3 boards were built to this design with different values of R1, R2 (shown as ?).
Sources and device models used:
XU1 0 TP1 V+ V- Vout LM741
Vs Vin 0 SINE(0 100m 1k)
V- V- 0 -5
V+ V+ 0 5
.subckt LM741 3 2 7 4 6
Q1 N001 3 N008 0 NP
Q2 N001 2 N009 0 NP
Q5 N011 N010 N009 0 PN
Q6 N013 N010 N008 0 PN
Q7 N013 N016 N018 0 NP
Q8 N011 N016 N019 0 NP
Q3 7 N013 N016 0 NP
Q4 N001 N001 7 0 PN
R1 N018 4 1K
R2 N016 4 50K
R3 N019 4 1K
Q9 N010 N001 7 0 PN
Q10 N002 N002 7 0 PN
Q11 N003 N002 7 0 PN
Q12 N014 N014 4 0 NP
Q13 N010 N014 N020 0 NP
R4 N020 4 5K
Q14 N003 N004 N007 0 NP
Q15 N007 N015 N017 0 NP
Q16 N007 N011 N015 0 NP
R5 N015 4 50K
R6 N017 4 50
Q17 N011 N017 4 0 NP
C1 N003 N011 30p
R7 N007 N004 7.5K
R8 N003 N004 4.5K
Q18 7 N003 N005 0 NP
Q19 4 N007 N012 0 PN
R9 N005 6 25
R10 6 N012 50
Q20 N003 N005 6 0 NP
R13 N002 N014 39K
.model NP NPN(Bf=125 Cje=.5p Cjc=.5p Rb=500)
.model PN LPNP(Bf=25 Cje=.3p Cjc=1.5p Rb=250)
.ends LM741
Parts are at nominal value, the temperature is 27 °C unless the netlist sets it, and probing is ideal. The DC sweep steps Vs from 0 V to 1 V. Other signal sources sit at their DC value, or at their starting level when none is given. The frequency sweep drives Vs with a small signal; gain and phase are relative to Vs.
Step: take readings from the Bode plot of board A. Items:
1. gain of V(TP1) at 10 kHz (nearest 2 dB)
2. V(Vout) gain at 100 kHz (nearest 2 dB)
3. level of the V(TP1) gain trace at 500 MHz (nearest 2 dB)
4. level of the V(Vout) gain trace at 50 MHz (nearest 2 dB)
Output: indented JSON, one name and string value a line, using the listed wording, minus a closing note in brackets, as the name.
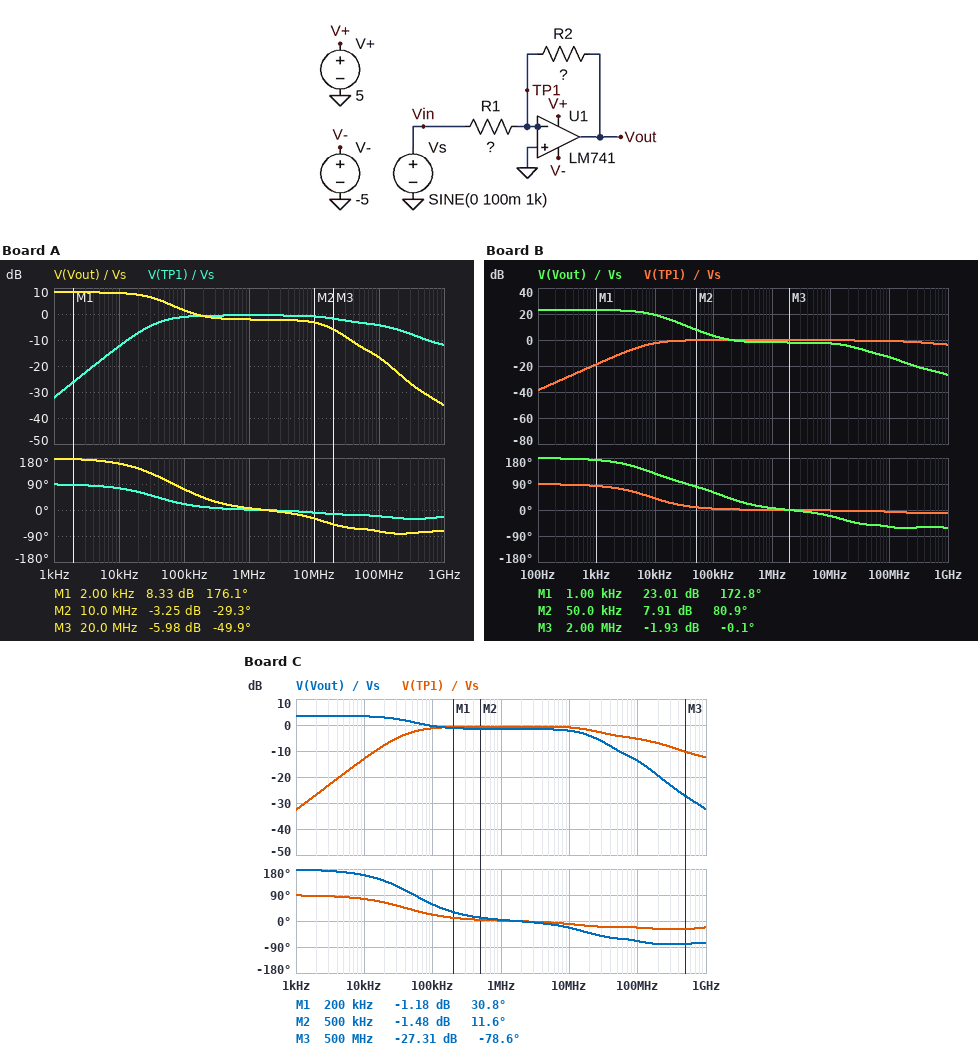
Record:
{
  "gain of V(TP1) at 10 kHz": "-12 dB",
  "V(Vout) gain at 100 kHz": "2 dB",
  "level of the V(TP1) gain trace at 500 MHz": "-10 dB",
  "level of the V(Vout) gain trace at 50 MHz": "-12 dB"
}
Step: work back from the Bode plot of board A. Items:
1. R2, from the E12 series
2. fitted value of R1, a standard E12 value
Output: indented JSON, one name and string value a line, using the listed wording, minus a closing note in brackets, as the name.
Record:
{
  "R2, from the E12 series": "4.7 kΩ",
  "fitted value of R1, a standard E12 value": "1.8 kΩ"
}
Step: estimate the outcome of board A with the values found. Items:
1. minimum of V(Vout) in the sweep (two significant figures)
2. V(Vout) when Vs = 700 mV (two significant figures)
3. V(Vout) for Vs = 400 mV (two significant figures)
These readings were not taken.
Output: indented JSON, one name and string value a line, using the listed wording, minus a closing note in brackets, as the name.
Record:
{
  "minimum of V(Vout) in the sweep": "-2.6 V",
  "V(Vout) when Vs = 700 mV": "-1.8 V",
  "V(Vout) for Vs = 400 mV": "-1.0 V"
}
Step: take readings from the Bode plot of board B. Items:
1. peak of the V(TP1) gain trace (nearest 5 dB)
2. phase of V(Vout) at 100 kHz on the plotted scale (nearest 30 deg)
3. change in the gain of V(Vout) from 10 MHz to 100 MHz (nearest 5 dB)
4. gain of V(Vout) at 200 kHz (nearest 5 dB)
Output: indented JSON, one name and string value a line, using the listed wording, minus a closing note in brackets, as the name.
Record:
{
  "peak of the V(TP1) gain trace": "0 dB",
  "phase of V(Vout) at 100 kHz on the plotted scale": "60 deg",
  "change in the gain of V(Vout) from 10 MHz to 100 MHz": "-10 dB",
  "gain of V(Vout) at 200 kHz": "0 dB"
}
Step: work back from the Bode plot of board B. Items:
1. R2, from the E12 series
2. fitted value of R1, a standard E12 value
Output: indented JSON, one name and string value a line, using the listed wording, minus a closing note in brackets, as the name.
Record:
{
  "R2, from the E12 series": "4.7 kΩ",
  "fitted value of R1, a standard E12 value": "330 Ω"
}
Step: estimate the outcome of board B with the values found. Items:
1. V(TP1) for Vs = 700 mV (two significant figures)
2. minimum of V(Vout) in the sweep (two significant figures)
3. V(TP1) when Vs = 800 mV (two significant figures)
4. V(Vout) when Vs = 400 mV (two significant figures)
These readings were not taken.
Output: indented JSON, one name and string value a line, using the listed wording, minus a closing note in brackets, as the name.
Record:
{
  "V(TP1) for Vs = 700 mV": "430 mV",
  "minimum of V(Vout) in the sweep": "-3.4 V",
  "V(TP1) when Vs = 800 mV": "520 mV",
  "V(Vout) when Vs = 400 mV": "-3.4 V"
}
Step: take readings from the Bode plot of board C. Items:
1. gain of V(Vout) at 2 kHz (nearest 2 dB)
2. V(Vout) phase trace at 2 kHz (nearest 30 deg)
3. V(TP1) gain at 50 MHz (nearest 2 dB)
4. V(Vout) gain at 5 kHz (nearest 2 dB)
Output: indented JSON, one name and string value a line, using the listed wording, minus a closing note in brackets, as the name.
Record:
{
  "gain of V(Vout) at 2 kHz": "4 dB",
  "V(Vout) phase trace at 2 kHz": "180 deg",
  "V(TP1) gain at 50 MHz": "-4 dB",
  "V(Vout) gain at 5 kHz": "4 dB"
}
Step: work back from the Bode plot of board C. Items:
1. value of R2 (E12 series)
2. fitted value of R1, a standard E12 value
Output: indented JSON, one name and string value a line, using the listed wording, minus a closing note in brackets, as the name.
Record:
{
  "value of R2": "2.7 kΩ",
  "fitted value of R1, a standard E12 value": "1.8 kΩ"
}
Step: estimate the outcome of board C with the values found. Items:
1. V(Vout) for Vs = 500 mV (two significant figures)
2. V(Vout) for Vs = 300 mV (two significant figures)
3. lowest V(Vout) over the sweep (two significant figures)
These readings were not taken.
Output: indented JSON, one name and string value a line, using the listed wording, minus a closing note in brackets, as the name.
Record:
{
  "V(Vout) for Vs = 500 mV": "-750 mV",
  "V(Vout) for Vs = 300 mV": "-450 mV",
  "lowest V(Vout) over the sweep": "-1.5 V"
}
